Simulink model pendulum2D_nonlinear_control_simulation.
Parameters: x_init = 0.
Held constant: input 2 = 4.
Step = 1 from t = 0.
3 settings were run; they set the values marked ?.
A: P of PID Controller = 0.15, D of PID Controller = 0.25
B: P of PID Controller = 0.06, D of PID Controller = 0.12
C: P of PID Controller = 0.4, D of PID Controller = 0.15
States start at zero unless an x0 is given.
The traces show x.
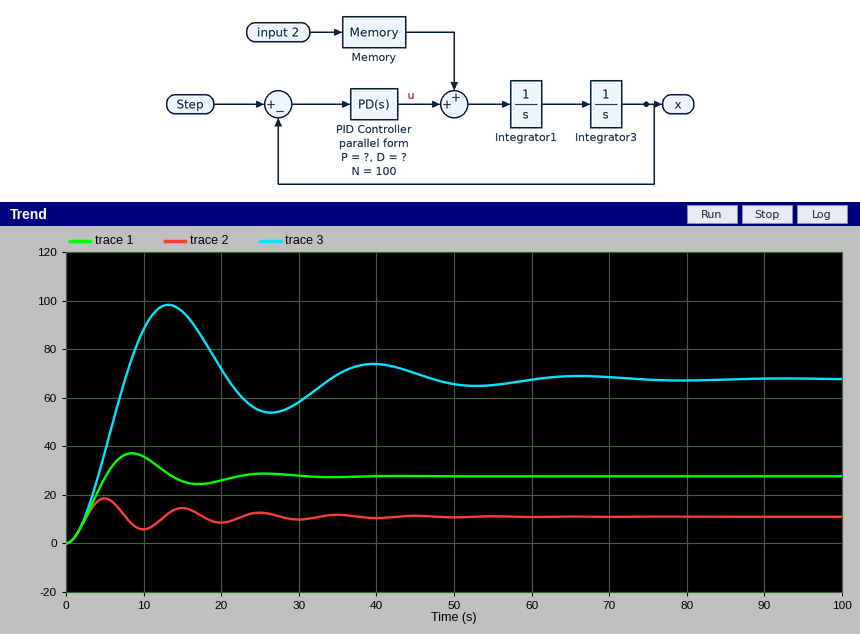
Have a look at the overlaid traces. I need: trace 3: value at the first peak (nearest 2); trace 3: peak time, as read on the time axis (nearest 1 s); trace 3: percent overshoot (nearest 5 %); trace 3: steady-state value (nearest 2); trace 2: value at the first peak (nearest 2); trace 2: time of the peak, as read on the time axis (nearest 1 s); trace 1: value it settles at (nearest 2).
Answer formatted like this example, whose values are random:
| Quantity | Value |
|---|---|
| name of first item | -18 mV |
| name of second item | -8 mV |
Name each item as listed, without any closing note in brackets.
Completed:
| Quantity | Value |
|---|---|
| trace 3: value at the first peak | 98 |
| trace 3: peak time, as read on the time axis | 13 s |
| trace 3: percent overshoot | 45 % |
| trace 3: steady-state value | 68 |
| trace 2: value at the first peak | 18 |
| trace 2: time of the peak, as read on the time axis | 5 s |
| trace 1: value it settles at | 28 |
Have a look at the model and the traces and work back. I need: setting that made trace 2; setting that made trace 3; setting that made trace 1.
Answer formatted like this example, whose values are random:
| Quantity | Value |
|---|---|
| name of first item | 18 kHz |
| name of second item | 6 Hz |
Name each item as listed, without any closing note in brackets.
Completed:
| Quantity | Value |
|---|---|
| setting that made trace 2 | C |
| setting that made trace 3 | B |
| setting that made trace 1 | A |
